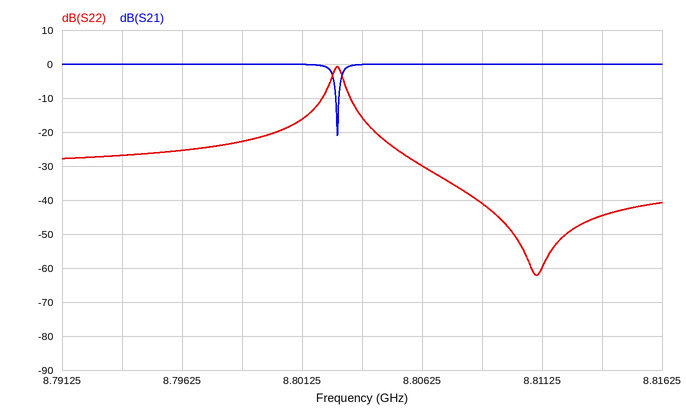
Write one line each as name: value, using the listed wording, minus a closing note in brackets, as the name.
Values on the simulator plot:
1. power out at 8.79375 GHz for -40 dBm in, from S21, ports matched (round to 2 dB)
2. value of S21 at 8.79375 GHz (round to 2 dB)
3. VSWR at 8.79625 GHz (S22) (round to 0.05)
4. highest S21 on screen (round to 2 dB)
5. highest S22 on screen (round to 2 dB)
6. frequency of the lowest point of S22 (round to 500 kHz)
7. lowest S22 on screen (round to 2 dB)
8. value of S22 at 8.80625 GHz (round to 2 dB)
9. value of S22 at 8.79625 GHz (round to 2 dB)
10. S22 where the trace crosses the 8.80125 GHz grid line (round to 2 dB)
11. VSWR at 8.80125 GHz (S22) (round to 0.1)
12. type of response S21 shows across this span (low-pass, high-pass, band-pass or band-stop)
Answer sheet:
power out at 8.79375 GHz for -40 dBm in, from S21, ports matched: -40 dBm
value of S21 at 8.79375 GHz: 0 dB
VSWR at 8.79625 GHz (S22): 1.10
highest S21 on screen: 0 dB
highest S22 on screen: 0 dB
frequency of the lowest point of S22: 8.8110 GHz
lowest S22 on screen: -62 dB
value of S22 at 8.80625 GHz: -30 dB
value of S22 at 8.79625 GHz: -26 dB
S22 where the trace crosses the 8.80125 GHz grid line: -16 dB
VSWR at 8.80125 GHz (S22): 1.4
type of response S21 shows across this span: band-stop
